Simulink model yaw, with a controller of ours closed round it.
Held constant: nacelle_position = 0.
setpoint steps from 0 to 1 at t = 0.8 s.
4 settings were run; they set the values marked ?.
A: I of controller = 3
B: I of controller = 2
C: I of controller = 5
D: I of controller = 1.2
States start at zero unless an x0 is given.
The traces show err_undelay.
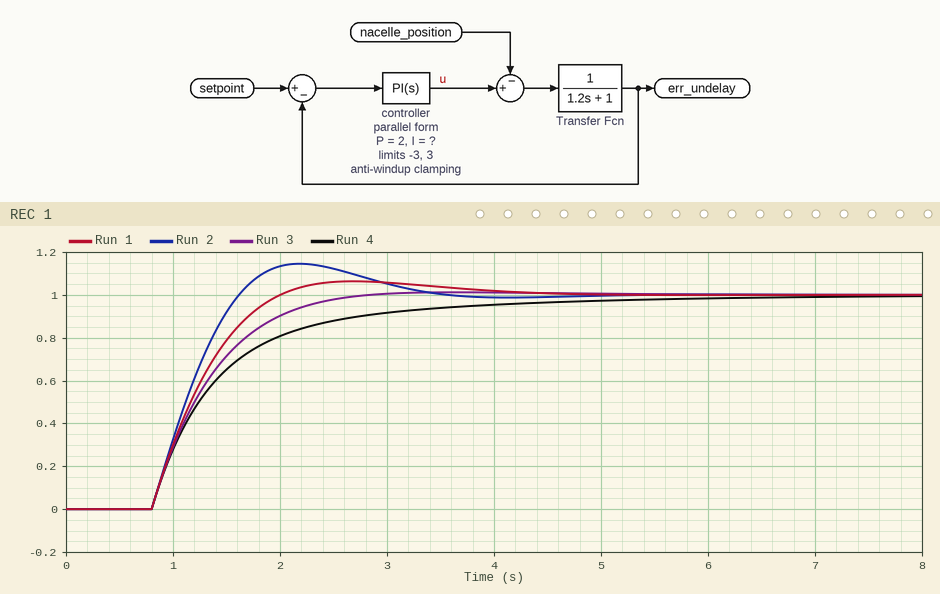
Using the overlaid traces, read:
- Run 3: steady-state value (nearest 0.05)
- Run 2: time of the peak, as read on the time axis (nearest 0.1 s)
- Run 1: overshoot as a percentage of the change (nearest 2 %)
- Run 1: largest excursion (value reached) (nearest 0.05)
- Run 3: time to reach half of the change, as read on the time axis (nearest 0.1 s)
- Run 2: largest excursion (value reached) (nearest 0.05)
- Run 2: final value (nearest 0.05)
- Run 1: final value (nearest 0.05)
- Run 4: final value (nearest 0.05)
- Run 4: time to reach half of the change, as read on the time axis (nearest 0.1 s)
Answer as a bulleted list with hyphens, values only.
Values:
- 1.00
- 2.2 s
- 6 %
- 1.05
- 1.2 s
- 1.15
- 1.00
- 1.00
- 1.00
- 1.2 s
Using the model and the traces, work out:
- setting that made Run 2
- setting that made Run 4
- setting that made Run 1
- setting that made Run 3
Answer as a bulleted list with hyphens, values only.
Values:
- C
- D
- A
- B
